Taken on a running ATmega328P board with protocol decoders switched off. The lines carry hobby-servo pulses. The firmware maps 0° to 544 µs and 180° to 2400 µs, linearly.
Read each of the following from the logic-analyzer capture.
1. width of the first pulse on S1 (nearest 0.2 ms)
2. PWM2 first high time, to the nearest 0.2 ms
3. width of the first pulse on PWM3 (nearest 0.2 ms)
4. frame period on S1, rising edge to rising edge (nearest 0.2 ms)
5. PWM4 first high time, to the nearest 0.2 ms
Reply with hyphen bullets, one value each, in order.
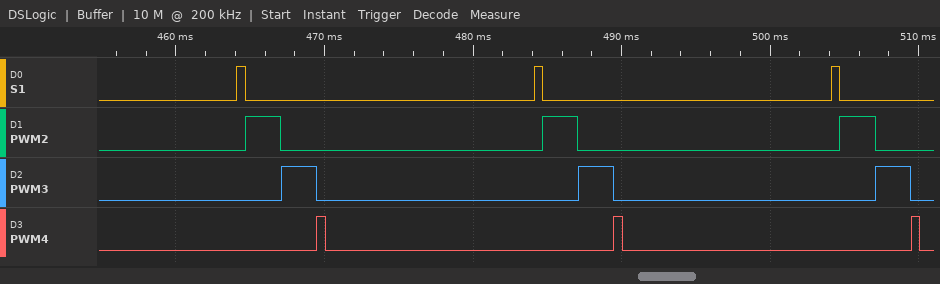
- 0.6 ms
- 2.4 ms
- 2.4 ms
- 20.0 ms
- 0.6 ms
